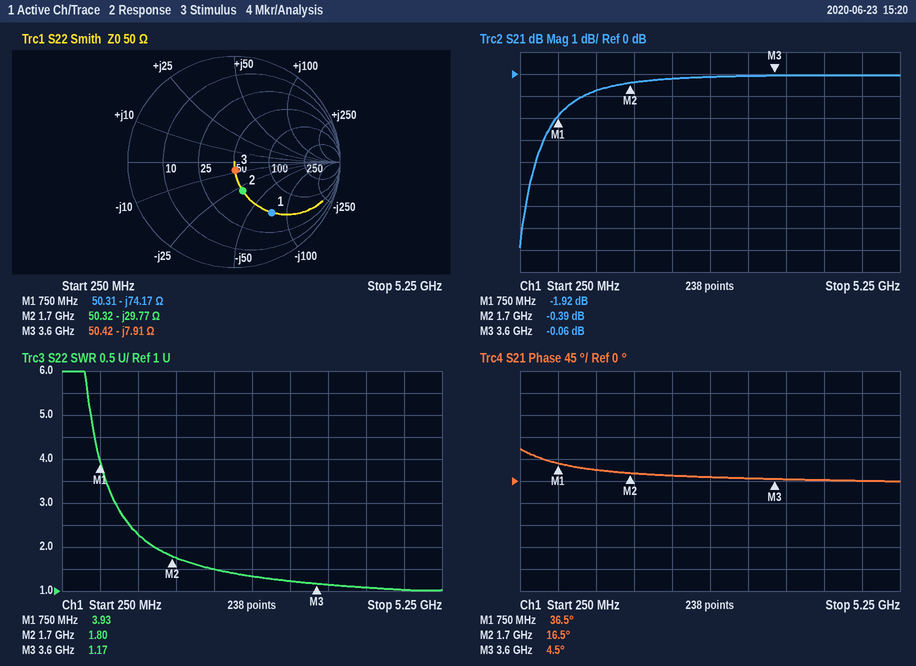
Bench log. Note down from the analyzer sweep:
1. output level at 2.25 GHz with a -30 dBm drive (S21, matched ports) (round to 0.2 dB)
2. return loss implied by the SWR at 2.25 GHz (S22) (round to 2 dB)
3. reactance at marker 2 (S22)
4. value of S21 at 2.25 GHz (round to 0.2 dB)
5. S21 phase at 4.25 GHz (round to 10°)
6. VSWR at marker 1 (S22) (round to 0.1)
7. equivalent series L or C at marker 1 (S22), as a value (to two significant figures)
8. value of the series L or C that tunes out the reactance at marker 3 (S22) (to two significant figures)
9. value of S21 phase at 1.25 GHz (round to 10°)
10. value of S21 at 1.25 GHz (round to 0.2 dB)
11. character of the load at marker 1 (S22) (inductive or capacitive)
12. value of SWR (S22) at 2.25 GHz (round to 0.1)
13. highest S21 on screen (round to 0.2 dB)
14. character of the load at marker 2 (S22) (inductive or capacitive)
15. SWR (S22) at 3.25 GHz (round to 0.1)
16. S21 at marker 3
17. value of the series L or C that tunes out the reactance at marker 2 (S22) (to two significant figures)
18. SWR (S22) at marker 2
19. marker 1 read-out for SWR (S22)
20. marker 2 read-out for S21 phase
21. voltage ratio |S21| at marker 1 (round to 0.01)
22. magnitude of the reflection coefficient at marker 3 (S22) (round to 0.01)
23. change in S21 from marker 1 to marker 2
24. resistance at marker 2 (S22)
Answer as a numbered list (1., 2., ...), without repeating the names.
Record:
1. -30.2 dBm
2. 14 dB
3. -29.77 Ω
4. -0.2 dB
5. 0°
6. 3.9
7. 2.9 pF
8. 350 pH
9. 20°
10. -0.8 dB
11. capacitive
12. 1.5
13. 0.0 dB
14. capacitive
15. 1.2
16. -0.06 dB
17. 2.8 nH
18. 1.80
19. 3.93
20. 16.5°
21. 0.80
22. 0.08
23. 1.53 dB
24. 50.32 Ω
